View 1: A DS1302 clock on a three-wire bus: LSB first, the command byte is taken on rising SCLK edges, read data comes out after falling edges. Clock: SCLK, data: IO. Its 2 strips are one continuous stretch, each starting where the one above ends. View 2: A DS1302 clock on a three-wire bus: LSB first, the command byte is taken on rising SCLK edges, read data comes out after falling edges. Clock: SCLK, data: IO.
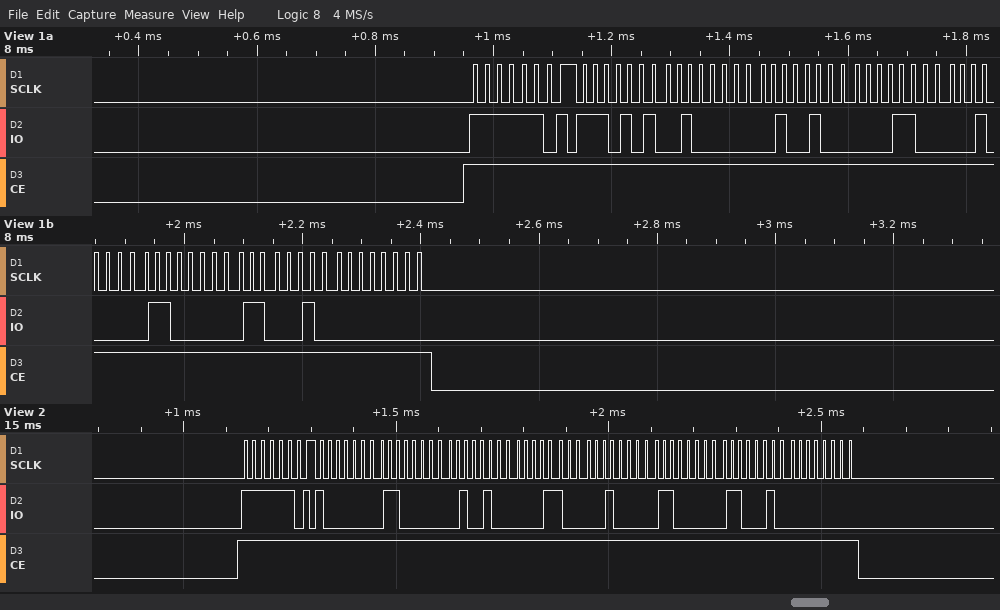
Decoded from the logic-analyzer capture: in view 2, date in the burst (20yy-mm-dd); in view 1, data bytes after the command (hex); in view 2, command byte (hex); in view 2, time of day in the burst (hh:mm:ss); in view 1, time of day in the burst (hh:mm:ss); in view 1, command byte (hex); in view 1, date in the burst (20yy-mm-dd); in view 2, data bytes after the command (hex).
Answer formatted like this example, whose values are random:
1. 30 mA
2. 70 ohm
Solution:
1. 2023-04-18
2. 57 02 12 18 04 03 23 00
3. 0xBF
4. 12:03:01
5. 12:02:57
6. 0xBF
7. 2023-04-18
8. 01 03 12 18 04 03 23 00
